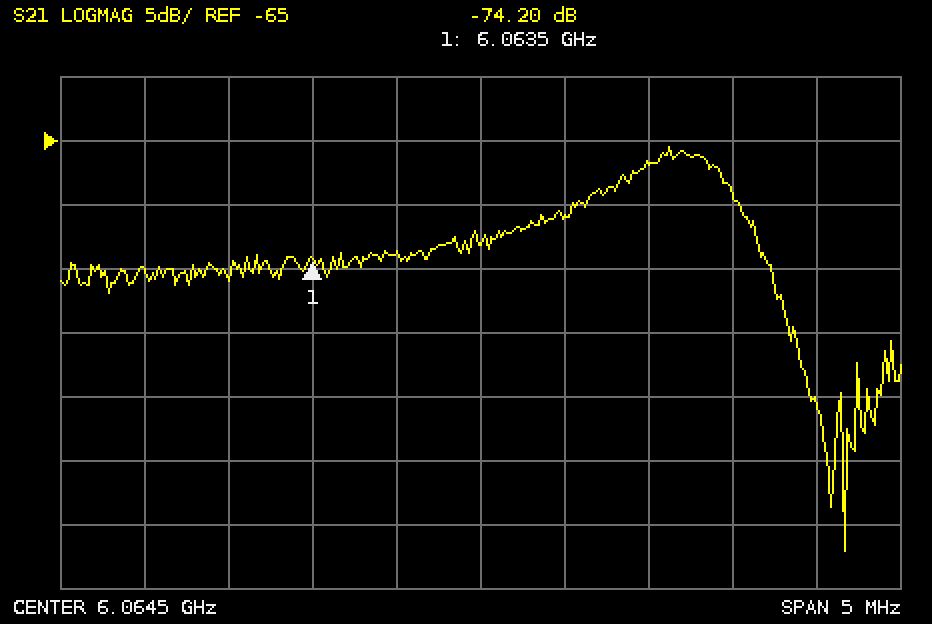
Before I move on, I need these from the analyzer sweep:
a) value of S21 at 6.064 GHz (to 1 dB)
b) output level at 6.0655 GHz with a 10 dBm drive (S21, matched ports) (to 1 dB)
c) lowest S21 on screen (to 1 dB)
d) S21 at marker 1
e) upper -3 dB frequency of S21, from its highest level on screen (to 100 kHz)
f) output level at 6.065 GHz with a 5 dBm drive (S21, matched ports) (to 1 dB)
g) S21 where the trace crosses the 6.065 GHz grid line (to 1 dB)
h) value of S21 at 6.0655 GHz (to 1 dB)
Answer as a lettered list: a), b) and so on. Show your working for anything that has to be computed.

a) -74 dB
b) 10 dBm + (-67 dB) = -57 dBm
c) -97 dB
d) -74.20 dB
e) 6.0660 GHz
f) 5 dBm + (-71 dB) = -66 dBm
g) -71 dB
h) -67 dB
